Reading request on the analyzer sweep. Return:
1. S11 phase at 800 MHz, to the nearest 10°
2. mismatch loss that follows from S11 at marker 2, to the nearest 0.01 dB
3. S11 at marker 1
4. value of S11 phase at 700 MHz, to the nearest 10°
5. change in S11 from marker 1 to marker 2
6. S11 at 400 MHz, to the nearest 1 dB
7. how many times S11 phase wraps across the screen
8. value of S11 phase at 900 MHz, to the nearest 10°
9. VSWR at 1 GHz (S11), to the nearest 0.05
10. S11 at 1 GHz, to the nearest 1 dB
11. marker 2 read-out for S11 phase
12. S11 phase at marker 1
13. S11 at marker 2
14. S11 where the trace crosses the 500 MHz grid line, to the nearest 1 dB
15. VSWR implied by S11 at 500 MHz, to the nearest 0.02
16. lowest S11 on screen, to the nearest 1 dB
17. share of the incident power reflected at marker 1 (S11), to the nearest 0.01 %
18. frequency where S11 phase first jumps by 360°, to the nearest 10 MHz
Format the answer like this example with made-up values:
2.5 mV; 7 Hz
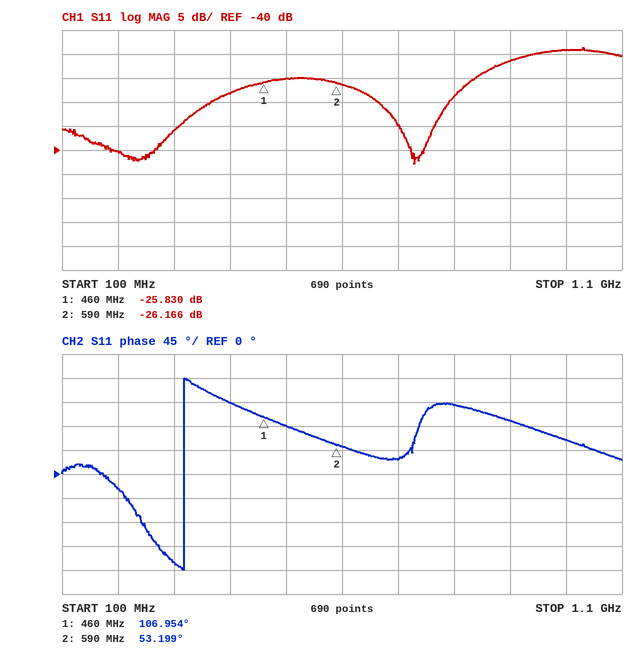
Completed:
130°; 0.01 dB; -25.830 dB; 30°; -0.336 dB; -28 dB; 1; 100°; 1.25; -19 dB; 53.199°; 106.954°; -26.166 dB; -25 dB; 1.12; -43 dB; 0.26 %; 320 MHz
